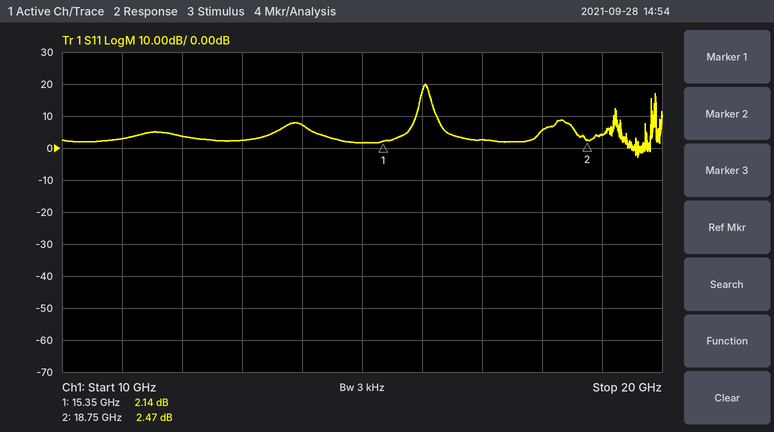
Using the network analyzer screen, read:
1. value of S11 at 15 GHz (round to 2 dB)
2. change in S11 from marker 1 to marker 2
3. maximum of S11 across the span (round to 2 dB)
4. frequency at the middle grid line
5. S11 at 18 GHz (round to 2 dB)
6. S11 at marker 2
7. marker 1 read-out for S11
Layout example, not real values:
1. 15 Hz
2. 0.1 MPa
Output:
1. 2 dB
2. 0.33 dB
3. 20 dB
4. 15 GHz
5. 6 dB
6. 2.47 dB
7. 2.14 dB
